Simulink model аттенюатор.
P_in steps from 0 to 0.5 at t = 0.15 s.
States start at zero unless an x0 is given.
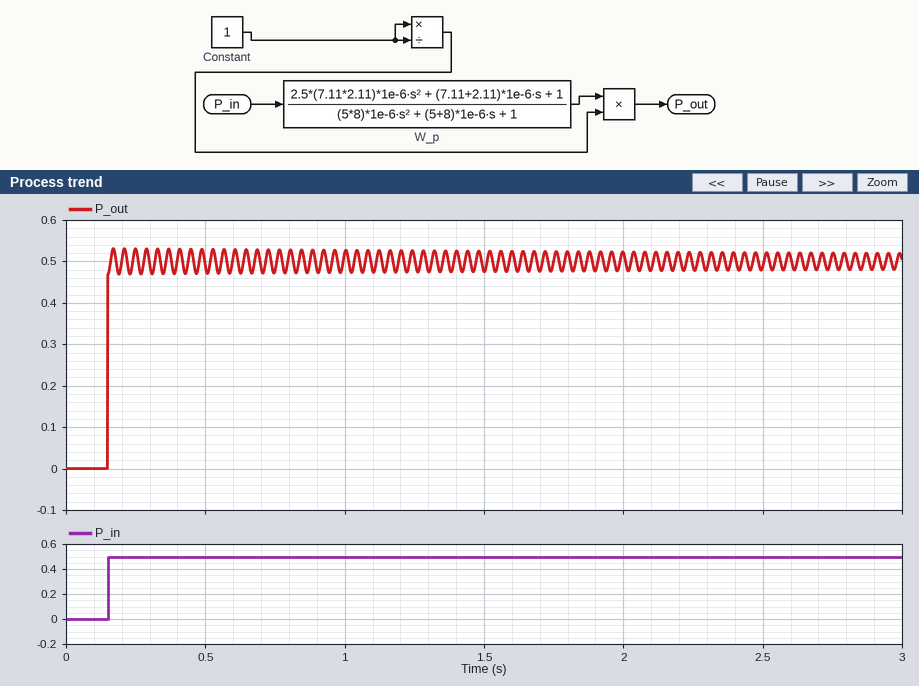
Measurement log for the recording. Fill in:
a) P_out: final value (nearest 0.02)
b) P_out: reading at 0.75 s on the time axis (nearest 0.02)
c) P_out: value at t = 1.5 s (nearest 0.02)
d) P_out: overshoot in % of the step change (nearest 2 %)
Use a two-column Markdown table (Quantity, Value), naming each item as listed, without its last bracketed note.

| Quantity | Value |
|---|---|
| P_out: final value | 0.50 |
| P_out: reading at 0.75 s on the time axis | 0.48 |
| P_out: value at t = 1.5 s | 0.48 |
| P_out: overshoot in % of the step change | 6 % |
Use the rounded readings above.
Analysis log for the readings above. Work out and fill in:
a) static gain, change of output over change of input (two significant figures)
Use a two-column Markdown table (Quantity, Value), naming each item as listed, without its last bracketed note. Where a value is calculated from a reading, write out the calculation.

| Quantity | Value |
|---|---|
| static gain, change of output over change of input | (0.5 - 0) / (0.5 - 0) = 1.0 |
